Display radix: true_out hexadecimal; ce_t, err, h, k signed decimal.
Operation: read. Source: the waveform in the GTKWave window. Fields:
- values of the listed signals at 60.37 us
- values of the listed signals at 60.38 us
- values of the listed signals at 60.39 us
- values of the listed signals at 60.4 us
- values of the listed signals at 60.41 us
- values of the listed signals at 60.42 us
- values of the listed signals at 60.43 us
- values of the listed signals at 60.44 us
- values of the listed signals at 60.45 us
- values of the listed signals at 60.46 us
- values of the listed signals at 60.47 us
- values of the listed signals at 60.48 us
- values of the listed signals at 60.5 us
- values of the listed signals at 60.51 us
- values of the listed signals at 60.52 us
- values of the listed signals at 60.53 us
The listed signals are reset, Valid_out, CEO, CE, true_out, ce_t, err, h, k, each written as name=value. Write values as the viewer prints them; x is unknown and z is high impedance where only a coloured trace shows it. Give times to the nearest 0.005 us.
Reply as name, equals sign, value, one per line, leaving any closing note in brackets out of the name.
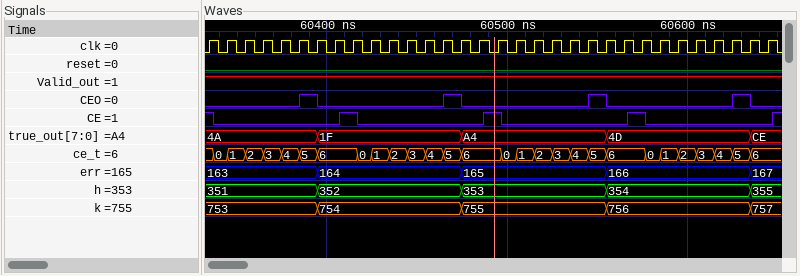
values of the listed signals at 60.37 us = reset=0, Valid_out=1, CEO=0, CE=0, true_out=4A, ce_t=3, err=163, h=351, k=753
values of the listed signals at 60.38 us = reset=0, Valid_out=1, CEO=0, CE=0, true_out=4A, ce_t=4, err=163, h=351, k=753
values of the listed signals at 60.39 us = reset=0, Valid_out=1, CEO=1, CE=0, true_out=4A, ce_t=5, err=163, h=351, k=753
values of the listed signals at 60.4 us = reset=0, Valid_out=1, CEO=0, CE=0, true_out=1F, ce_t=6, err=164, h=352, k=754
values of the listed signals at 60.41 us = reset=0, Valid_out=1, CEO=0, CE=1, true_out=1F, ce_t=6, err=164, h=352, k=754
values of the listed signals at 60.42 us = reset=0, Valid_out=1, CEO=0, CE=0, true_out=1F, ce_t=0, err=164, h=352, k=754
values of the listed signals at 60.43 us = reset=0, Valid_out=1, CEO=0, CE=0, true_out=1F, ce_t=1, err=164, h=352, k=754
values of the listed signals at 60.44 us = reset=0, Valid_out=1, CEO=0, CE=0, true_out=1F, ce_t=2, err=164, h=352, k=754
values of the listed signals at 60.45 us = reset=0, Valid_out=1, CEO=0, CE=0, true_out=1F, ce_t=3, err=164, h=352, k=754
values of the listed signals at 60.46 us = reset=0, Valid_out=1, CEO=0, CE=0, true_out=1F, ce_t=4, err=164, h=352, k=754
values of the listed signals at 60.47 us = reset=0, Valid_out=1, CEO=1, CE=0, true_out=1F, ce_t=5, err=164, h=352, k=754
values of the listed signals at 60.48 us = reset=0, Valid_out=1, CEO=0, CE=0, true_out=A4, ce_t=6, err=165, h=353, k=755
values of the listed signals at 60.5 us = reset=0, Valid_out=1, CEO=0, CE=0, true_out=A4, ce_t=0, err=165, h=353, k=755
values of the listed signals at 60.51 us = reset=0, Valid_out=1, CEO=0, CE=0, true_out=A4, ce_t=1, err=165, h=353, k=755
values of the listed signals at 60.52 us = reset=0, Valid_out=1, CEO=0, CE=0, true_out=A4, ce_t=2, err=165, h=353, k=755
values of the listed signals at 60.53 us = reset=0, Valid_out=1, CEO=0, CE=0, true_out=A4, ce_t=3, err=165, h=353, k=755
